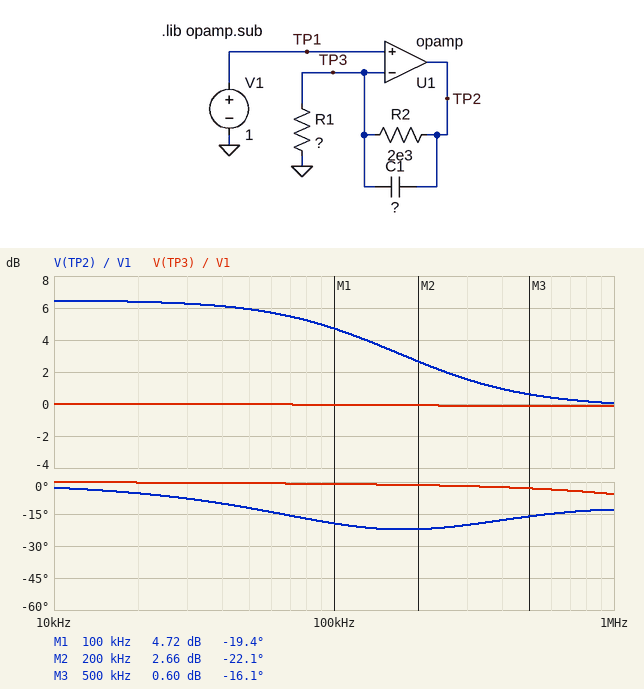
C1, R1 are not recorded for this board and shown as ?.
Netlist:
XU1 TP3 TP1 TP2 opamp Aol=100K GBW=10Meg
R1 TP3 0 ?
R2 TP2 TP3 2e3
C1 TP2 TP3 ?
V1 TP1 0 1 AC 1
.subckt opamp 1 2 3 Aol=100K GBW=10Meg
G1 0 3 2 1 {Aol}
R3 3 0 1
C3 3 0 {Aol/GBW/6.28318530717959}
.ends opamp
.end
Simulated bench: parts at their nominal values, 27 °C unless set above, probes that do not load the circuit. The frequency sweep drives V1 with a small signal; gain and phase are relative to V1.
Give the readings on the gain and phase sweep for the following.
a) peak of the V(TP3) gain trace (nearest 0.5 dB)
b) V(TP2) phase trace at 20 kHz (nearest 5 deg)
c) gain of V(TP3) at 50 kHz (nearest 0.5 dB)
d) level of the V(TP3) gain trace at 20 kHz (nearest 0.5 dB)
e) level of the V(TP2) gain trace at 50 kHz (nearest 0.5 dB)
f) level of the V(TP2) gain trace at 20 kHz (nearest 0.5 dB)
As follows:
0 dB
-5 deg
0 dB
0 dB
6.0 dB
6.5 dB
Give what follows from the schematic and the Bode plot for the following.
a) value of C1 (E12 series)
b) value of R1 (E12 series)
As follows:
680 pF
1.8 kΩ
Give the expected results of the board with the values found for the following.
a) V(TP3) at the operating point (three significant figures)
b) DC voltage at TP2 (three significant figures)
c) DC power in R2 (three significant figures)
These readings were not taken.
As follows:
1.00 V
2.11 V
617 µW
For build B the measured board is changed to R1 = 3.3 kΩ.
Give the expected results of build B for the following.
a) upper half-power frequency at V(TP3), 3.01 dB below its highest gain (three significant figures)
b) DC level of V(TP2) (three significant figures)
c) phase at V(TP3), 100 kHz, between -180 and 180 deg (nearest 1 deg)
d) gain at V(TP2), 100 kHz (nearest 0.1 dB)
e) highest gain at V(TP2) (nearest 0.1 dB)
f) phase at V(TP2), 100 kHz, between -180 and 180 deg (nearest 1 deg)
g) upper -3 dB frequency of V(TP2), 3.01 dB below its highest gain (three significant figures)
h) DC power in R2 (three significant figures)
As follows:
9.93 MHz
1.61 V
-1 deg
2.8 dB
4.1 dB
-13 deg
239 kHz
184 µW
